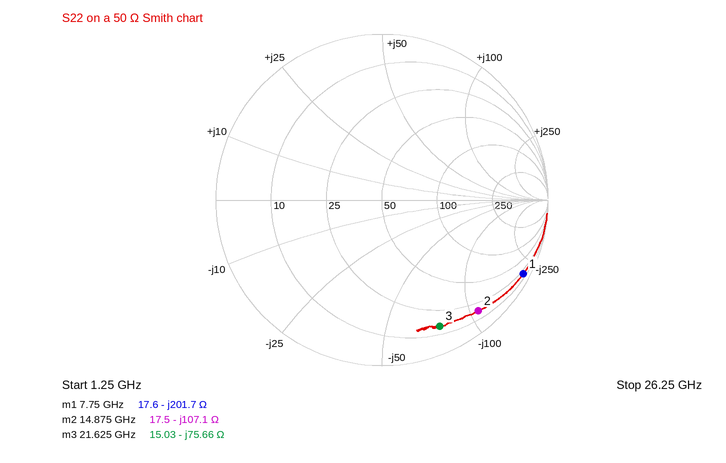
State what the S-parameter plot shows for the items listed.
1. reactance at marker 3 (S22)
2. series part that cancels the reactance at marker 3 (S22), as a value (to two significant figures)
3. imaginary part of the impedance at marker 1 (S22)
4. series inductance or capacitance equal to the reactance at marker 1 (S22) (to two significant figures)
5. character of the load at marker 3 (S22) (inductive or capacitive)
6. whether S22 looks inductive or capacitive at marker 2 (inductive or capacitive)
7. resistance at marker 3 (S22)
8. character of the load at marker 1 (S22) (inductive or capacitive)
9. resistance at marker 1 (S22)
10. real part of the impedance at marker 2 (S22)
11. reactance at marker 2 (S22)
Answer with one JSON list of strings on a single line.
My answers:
["-75.66 Ω", "560 pH", "-201.7 Ω", "100 fF", "capacitive", "capacitive", "15.03 Ω", "capacitive", "17.6 Ω", "17.5 Ω", "-107.1 Ω"]
